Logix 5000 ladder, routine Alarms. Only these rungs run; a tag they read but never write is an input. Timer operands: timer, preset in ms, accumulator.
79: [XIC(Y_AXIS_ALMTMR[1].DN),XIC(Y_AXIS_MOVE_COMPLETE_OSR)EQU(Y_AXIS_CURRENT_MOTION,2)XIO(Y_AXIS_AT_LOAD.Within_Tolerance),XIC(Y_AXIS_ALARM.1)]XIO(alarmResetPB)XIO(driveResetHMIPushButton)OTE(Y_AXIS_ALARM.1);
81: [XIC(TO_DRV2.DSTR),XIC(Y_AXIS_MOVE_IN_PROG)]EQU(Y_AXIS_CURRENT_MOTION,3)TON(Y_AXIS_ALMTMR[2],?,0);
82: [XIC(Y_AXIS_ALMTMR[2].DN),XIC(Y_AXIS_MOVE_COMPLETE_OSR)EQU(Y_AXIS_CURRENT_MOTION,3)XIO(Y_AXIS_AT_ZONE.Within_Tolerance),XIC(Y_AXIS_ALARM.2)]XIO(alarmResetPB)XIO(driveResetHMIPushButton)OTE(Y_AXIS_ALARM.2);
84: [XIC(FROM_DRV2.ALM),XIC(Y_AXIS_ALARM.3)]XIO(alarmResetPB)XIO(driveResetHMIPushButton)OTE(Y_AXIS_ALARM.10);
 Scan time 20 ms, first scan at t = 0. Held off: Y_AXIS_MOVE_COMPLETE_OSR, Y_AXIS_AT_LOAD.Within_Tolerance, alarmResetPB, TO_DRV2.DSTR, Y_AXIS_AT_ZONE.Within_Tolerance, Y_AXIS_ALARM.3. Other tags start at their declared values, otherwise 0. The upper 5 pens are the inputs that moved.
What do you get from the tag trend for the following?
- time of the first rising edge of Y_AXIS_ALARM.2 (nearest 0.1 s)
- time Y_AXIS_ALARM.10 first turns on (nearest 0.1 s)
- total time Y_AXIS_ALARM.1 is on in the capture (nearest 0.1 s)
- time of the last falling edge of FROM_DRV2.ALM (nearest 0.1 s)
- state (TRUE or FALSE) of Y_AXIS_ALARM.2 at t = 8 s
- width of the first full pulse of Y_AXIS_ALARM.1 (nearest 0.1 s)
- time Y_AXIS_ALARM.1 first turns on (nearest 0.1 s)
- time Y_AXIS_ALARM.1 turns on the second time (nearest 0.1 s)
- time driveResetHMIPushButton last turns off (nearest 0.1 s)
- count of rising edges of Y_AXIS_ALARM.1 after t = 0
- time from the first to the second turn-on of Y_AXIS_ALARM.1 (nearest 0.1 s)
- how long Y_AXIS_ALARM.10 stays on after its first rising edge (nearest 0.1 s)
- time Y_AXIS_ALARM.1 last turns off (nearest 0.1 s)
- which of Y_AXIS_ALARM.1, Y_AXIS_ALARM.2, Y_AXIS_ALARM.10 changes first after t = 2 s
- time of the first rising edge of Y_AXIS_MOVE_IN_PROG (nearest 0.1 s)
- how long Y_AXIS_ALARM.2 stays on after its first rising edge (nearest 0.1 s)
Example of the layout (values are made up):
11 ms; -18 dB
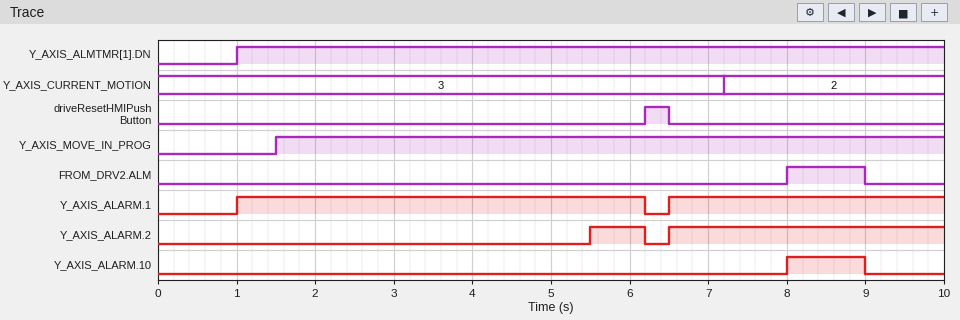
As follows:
5.5 s; 8.0 s; 8.7 s; 9.0 s; TRUE; 5.2 s; 1.0 s; 6.5 s; 6.5 s; 2; 5.5 s; 1.0 s; 6.2 s; Y_AXIS_ALARM.2; 1.5 s; 0.7 s
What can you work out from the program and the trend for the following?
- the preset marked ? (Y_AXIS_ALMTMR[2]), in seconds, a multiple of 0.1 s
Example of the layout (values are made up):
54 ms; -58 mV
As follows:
4.0 s
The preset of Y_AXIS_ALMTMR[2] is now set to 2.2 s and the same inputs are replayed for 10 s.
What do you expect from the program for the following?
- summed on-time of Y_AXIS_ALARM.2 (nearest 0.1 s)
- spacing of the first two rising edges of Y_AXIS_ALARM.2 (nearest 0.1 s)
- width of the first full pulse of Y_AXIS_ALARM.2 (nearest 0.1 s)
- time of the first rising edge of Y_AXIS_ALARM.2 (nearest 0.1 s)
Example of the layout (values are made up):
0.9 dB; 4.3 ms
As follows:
6.0 s; 2.8 s; 2.5 s; 3.7 s
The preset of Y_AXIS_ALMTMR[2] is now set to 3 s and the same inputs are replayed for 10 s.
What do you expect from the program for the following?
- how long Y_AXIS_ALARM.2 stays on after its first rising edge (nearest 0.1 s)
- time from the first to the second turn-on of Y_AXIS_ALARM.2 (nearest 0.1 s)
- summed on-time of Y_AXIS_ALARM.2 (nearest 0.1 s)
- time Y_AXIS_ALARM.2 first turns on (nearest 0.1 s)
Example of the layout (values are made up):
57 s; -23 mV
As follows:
1.7 s; 2.0 s; 5.2 s; 4.5 s
